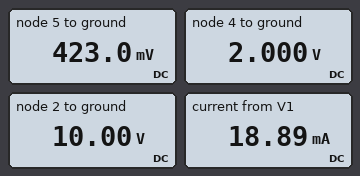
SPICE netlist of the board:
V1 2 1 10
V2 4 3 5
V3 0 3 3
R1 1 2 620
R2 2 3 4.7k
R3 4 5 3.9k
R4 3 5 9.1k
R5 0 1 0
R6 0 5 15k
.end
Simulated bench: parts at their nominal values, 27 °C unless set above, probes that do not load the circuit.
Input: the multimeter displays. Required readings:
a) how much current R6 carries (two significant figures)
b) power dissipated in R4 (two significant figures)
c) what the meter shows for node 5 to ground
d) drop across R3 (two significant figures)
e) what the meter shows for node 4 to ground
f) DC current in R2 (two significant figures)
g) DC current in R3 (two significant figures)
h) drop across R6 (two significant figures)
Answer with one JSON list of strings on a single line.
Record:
["28 µA", "1.3 mW", "423.0 mV", "1.6 V", "2.000 V", "2.8 mA", "400 µA", "420 mV"]
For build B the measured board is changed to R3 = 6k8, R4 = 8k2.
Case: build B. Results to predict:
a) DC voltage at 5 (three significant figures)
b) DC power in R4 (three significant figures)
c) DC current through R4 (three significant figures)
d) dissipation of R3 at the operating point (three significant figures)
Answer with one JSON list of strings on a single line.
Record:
["-214 mV", "947 µW", "340 µA", "721 µW"]
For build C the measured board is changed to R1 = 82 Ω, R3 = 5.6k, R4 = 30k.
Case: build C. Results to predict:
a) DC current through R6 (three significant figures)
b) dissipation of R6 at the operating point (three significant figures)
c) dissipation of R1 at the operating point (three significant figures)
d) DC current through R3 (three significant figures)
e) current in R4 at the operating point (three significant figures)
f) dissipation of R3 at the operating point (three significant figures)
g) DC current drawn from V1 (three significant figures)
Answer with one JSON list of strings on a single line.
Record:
["61.5 µA", "56.8 µW", "1.22 W", "192 µA", "131 µA", "207 µW", "125 mA"]
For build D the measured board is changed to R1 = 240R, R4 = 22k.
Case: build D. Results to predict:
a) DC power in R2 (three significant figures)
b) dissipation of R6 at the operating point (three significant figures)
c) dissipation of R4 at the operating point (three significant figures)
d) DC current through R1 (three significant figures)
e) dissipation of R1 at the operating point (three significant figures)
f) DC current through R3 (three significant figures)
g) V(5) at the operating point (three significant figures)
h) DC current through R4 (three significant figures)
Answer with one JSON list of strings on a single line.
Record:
["36.0 mW", "69.6 µW", "735 µW", "41.7 mA", "417 mW", "251 µA", "1.02 V", "183 µA"]
